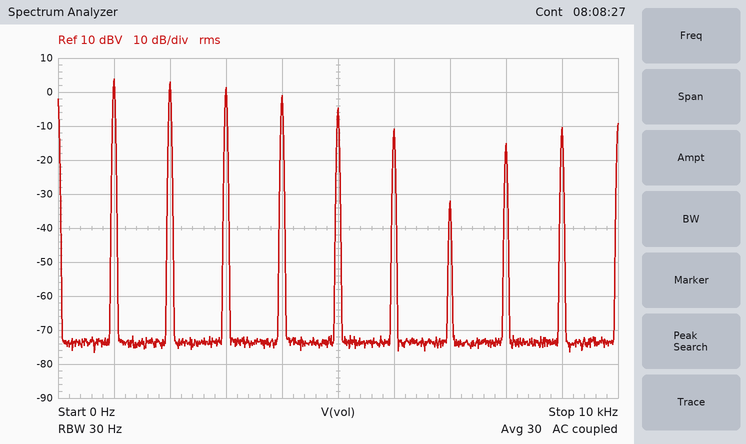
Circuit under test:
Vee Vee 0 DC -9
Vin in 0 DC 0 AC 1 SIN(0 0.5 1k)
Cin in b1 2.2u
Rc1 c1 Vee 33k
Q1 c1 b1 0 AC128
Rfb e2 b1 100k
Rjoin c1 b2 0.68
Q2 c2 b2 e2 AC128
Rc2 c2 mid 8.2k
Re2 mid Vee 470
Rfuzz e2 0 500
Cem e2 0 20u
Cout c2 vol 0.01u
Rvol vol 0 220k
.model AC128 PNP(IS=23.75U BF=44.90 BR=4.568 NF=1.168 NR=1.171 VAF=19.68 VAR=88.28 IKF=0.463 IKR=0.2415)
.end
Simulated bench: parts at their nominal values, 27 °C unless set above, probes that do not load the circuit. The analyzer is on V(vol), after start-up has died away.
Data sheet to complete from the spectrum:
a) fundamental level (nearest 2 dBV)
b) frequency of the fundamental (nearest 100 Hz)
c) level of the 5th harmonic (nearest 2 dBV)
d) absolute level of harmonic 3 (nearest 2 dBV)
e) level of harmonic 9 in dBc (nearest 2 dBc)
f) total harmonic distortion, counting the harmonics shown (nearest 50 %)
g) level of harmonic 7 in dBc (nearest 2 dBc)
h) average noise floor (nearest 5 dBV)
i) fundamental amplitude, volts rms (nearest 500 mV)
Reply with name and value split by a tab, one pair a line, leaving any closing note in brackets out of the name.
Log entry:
fundamental level	4 dBV
frequency of the fundamental	1.0 kHz
level of the 5th harmonic	-4 dBV
absolute level of harmonic 3	2 dBV
level of harmonic 9 in dBc	-14 dBc
total harmonic distortion, counting the harmonics shown	150 %
level of harmonic 7 in dBc	-36 dBc
average noise floor	-75 dBV
fundamental amplitude, volts rms	1.5 V
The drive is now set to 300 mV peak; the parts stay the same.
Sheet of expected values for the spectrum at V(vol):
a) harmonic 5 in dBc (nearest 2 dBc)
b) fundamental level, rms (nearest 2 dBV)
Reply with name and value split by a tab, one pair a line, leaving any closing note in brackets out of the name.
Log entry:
harmonic 5 in dBc	-14 dBc
fundamental level, rms	6 dBV
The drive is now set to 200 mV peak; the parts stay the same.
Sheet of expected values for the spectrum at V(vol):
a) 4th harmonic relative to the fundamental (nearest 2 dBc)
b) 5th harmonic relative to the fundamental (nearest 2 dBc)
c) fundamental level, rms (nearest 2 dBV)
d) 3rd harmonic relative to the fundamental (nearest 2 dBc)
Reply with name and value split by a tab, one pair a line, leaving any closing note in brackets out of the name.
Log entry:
4th harmonic relative to the fundamental	-10 dBc
5th harmonic relative to the fundamental	-24 dBc
fundamental level, rms	6 dBV
3rd harmonic relative to the fundamental	-4 dBc
